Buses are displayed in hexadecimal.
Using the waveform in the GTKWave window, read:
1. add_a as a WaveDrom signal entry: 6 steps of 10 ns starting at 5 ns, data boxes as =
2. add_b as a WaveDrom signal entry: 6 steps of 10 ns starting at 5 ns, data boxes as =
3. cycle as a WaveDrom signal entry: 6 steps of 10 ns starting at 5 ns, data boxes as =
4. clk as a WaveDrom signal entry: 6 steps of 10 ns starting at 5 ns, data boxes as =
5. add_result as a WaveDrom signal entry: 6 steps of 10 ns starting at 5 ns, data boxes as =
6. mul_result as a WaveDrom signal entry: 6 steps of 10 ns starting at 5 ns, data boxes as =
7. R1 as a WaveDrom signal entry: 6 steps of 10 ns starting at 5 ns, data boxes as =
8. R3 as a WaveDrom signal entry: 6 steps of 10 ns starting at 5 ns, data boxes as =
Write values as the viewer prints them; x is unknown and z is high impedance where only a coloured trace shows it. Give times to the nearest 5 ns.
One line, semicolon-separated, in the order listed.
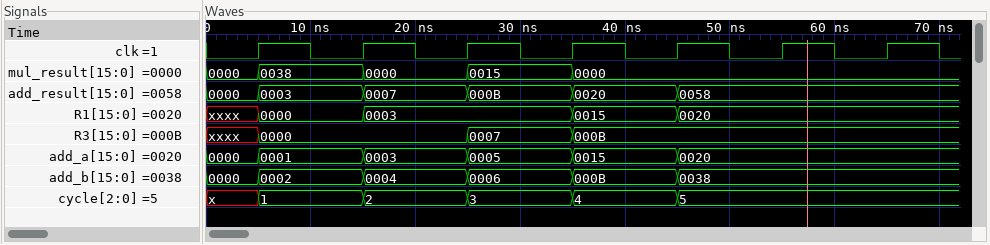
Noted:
{name: 'add_a', wave: '=====.', data: '0001 0003 0005 0015 0020'}; {name: 'add_b', wave: '=====.', data: '0002 0004 0006 000B 0038'}; {name: 'cycle', wave: '=====.', data: '1 2 3 4 5'}; {name: 'clk', wave: 'p.....'}; {name: 'add_result', wave: '=====.', data: '0003 0007 000B 0020 0058'}; {name: 'mul_result', wave: '====..', data: '0038 0000 0015 0000'}; {name: 'R1', wave: '==.==.', data: '0000 0003 0015 0020'}; {name: 'R3', wave: '=.==..', data: '0000 0007 000B'}
